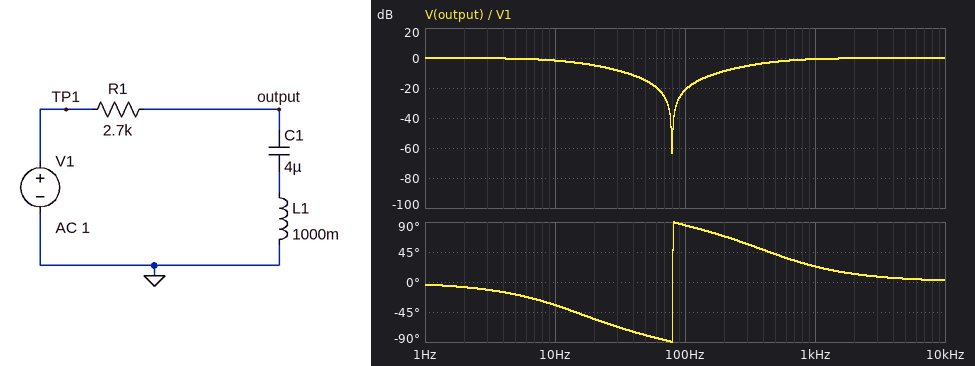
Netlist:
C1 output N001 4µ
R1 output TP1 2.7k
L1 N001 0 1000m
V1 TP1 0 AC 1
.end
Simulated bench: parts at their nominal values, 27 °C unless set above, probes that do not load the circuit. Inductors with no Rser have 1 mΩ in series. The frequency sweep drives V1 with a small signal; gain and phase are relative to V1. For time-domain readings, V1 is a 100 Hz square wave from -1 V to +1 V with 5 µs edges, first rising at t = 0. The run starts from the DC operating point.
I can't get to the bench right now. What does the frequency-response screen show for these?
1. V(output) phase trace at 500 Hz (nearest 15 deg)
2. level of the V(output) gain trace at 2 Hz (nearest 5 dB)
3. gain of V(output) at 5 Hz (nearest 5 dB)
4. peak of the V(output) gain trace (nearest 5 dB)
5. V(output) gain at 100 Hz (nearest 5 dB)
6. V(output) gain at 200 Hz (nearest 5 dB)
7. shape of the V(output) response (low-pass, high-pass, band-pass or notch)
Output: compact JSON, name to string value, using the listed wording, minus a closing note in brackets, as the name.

{"V(output) phase trace at 500 Hz": "45 deg", "level of the V(output) gain trace at 2 Hz": "0 dB", "gain of V(output) at 5 Hz": "0 dB", "peak of the V(output) gain trace": "0 dB", "V(output) gain at 100 Hz": "-20 dB", "V(output) gain at 200 Hz": "-10 dB", "shape of the V(output) response": "notch"}
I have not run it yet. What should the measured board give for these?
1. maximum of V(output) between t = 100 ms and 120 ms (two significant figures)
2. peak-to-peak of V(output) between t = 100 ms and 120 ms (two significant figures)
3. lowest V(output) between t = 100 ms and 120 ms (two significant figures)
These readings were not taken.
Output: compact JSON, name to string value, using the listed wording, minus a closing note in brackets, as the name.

{"maximum of V(output) between t = 100 ms and 120 ms": "1.8 V", "peak-to-peak of V(output) between t = 100 ms and 120 ms": "3.6 V", "lowest V(output) between t = 100 ms and 120 ms": "-1.8 V"}
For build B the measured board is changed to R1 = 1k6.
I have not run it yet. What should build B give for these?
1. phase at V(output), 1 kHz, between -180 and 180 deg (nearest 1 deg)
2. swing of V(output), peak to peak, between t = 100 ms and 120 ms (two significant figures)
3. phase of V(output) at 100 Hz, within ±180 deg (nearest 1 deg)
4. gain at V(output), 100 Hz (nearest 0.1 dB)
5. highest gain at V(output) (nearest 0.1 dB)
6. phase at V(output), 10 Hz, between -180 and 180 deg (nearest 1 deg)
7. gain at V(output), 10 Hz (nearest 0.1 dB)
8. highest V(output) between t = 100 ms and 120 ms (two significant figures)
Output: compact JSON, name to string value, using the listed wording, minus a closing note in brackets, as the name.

{"phase at V(output), 1 kHz, between -180 and 180 deg": "14 deg", "swing of V(output), peak to peak, between t = 100 ms and 120 ms": "3.5 V", "phase of V(output) at 100 Hz, within ±180 deg": "82 deg", "gain at V(output), 100 Hz": "-16.9 dB", "highest gain at V(output)": "0 dB", "phase at V(output), 10 Hz, between -180 and 180 deg": "-22 deg", "gain at V(output), 10 Hz": "-0.7 dB", "highest V(output) between t = 100 ms and 120 ms": "1.7 V"}
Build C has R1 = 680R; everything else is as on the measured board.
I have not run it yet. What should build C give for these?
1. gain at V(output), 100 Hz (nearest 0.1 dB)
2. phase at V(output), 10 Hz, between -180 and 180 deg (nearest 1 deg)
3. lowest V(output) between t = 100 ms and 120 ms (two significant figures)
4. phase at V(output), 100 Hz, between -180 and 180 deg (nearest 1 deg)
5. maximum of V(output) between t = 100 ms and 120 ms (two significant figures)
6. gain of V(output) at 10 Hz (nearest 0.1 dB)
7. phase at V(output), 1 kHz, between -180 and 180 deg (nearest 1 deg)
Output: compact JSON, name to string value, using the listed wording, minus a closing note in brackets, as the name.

{"gain at V(output), 100 Hz": "-9.9 dB", "phase at V(output), 10 Hz, between -180 and 180 deg": "-10 deg", "lowest V(output) between t = 100 ms and 120 ms": "-1.7 V", "phase at V(output), 100 Hz, between -180 and 180 deg": "71 deg", "maximum of V(output) between t = 100 ms and 120 ms": "1.7 V", "gain of V(output) at 10 Hz": "-0.1 dB", "phase at V(output), 1 kHz, between -180 and 180 deg": "6 deg"}
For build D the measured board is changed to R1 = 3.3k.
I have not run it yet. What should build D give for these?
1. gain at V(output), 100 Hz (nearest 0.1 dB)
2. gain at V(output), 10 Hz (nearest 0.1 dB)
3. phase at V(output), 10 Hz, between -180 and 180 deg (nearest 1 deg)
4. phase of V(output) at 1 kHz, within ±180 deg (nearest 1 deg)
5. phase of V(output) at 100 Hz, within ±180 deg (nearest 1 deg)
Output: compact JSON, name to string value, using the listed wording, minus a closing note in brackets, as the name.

{"gain at V(output), 100 Hz": "-23.1 dB", "gain at V(output), 10 Hz": "-2.3 dB", "phase at V(output), 10 Hz, between -180 and 180 deg": "-40 deg", "phase of V(output) at 1 kHz, within ±180 deg": "28 deg", "phase of V(output) at 100 Hz, within ±180 deg": "86 deg"}
